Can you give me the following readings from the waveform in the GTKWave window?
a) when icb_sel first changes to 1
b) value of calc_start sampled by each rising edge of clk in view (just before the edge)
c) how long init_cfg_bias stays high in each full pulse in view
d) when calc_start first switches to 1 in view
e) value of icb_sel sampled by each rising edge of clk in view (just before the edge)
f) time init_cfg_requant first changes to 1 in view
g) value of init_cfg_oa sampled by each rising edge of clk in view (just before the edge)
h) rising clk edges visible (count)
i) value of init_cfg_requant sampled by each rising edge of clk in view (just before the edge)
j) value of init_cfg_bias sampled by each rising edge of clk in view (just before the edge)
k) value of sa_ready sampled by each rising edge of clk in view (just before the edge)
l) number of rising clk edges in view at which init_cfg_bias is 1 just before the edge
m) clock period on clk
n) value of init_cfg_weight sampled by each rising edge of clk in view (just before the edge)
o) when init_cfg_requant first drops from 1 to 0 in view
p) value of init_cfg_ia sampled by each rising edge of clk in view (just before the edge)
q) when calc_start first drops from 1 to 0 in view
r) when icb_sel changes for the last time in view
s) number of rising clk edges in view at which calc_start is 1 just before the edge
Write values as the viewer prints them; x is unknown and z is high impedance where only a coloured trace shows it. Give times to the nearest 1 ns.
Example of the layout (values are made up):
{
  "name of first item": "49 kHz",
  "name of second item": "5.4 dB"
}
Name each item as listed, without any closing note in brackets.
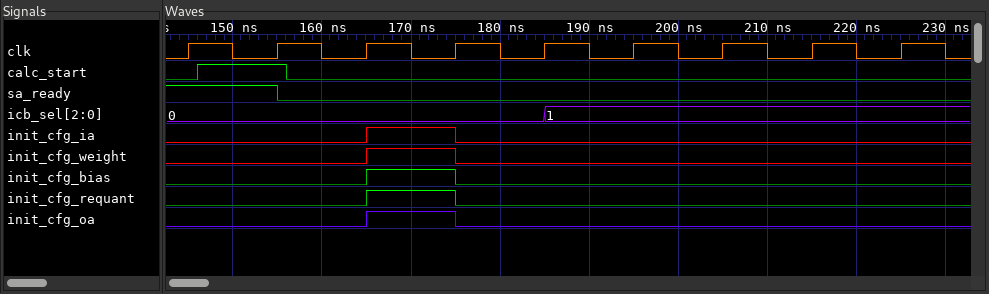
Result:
{
  "when icb_sel first changes to 1": "185 ns",
  "value of calc_start sampled by each rising edge of clk in view": "0 1 0 0 0 0 0 0 0",
  "how long init_cfg_bias stays high in each full pulse in view": "10 ns",
  "when calc_start first switches to 1 in view": "146 ns",
  "value of icb_sel sampled by each rising edge of clk in view": "0, 0, 0, 0, 0, 1, 1, 1, 1",
  "time init_cfg_requant first changes to 1 in view": "165 ns",
  "value of init_cfg_oa sampled by each rising edge of clk in view": "0 0 0 1 0 0 0 0 0",
  "rising clk edges visible": "9",
  "value of init_cfg_requant sampled by each rising edge of clk in view": "0 0 0 1 0 0 0 0 0",
  "value of init_cfg_bias sampled by each rising edge of clk in view": "0 0 0 1 0 0 0 0 0",
  "value of sa_ready sampled by each rising edge of clk in view": "1 1 0 0 0 0 0 0 0",
  "number of rising clk edges in view at which init_cfg_bias is 1 just before the edge": "1",
  "clock period on clk": "10 ns",
  "value of init_cfg_weight sampled by each rising edge of clk in view": "0 0 0 1 0 0 0 0 0",
  "when init_cfg_requant first drops from 1 to 0 in view": "175 ns",
  "value of init_cfg_ia sampled by each rising edge of clk in view": "0 0 0 1 0 0 0 0 0",
  "when calc_start first drops from 1 to 0 in view": "156 ns",
  "when icb_sel changes for the last time in view": "185 ns",
  "number of rising clk edges in view at which calc_start is 1 just before the edge": "1"
}
